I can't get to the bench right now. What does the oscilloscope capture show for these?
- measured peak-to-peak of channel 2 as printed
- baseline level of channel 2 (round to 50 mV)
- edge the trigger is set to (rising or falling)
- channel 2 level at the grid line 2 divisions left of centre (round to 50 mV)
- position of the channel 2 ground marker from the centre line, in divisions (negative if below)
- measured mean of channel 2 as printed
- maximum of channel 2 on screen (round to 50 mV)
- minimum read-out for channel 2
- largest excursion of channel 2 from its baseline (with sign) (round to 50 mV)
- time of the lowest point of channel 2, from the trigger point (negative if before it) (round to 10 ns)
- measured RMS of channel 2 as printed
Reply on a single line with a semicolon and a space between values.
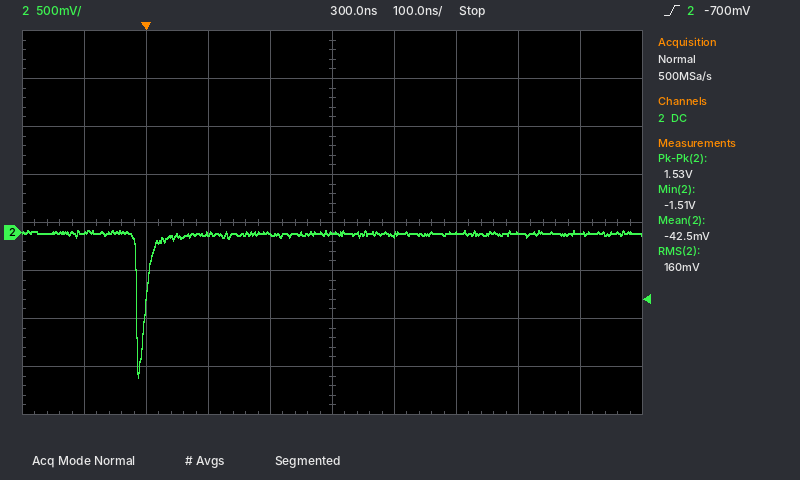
1.53 V; 0 mV; rising; 0 mV; -0.2 div; -42.5 mV; 0 mV; -1.51 V; -1.50 V; -10 ns; 160 mV
